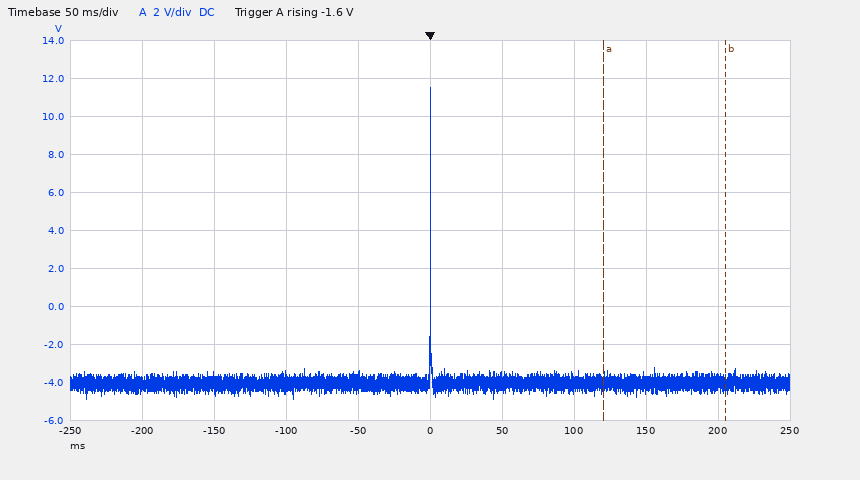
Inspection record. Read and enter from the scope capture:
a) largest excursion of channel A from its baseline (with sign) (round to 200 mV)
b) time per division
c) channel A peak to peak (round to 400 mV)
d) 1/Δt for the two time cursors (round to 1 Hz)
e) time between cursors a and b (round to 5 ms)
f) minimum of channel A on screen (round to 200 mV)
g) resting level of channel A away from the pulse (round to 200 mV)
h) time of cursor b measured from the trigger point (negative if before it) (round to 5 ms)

+15.6 V
50 ms
16.4 V
12 Hz
85 ms
-4.8 V
-4.0 V
+205 ms
